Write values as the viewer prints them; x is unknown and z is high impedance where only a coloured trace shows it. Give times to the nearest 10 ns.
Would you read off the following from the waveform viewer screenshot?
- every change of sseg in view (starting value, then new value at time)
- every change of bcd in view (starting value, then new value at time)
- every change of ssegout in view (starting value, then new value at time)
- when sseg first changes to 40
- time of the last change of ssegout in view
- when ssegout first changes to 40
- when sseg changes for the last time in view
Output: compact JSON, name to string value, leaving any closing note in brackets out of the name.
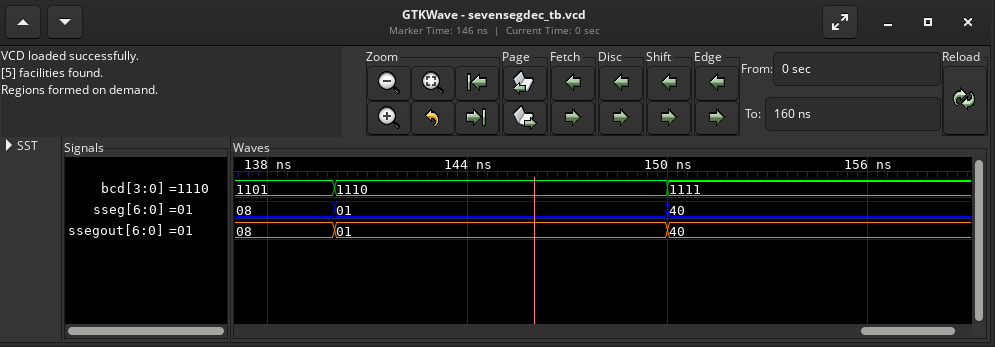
{"every change of sseg in view": "08, 01 at 140 ns, 40 at 150 ns", "every change of bcd in view": "1101, 1110 at 140 ns, 1111 at 150 ns", "every change of ssegout in view": "08, 01 at 140 ns, 40 at 150 ns", "when sseg first changes to 40": "150 ns", "time of the last change of ssegout in view": "150 ns", "when ssegout first changes to 40": "150 ns", "when sseg changes for the last time in view": "150 ns"}
